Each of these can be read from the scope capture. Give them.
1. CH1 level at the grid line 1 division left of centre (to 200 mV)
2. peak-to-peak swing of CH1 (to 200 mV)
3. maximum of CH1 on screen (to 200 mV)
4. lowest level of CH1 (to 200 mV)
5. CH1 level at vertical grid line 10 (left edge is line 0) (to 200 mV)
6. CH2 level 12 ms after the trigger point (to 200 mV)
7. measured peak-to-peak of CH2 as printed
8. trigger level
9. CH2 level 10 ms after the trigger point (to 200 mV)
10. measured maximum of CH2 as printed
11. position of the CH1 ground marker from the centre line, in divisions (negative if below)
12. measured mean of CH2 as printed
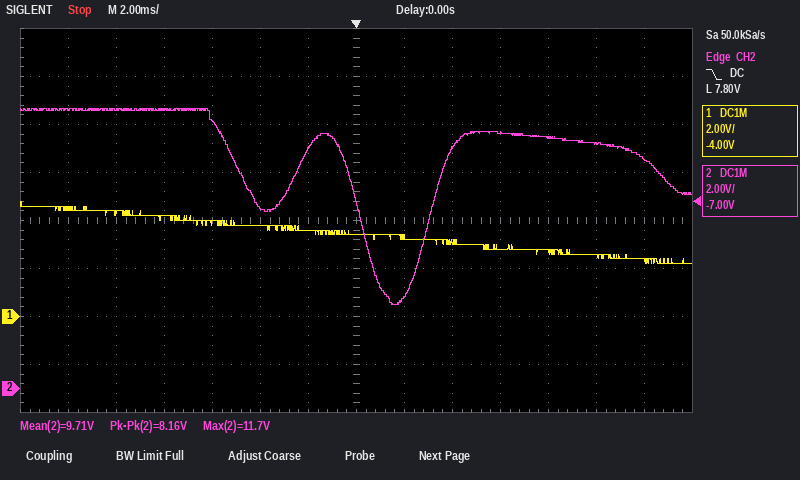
3.6 V
2.6 V
4.8 V
2.2 V
2.8 V
9.6 V
8.16 V
7.80 V
10.2 V
11.7 V
-2.0 div
9.71 V
